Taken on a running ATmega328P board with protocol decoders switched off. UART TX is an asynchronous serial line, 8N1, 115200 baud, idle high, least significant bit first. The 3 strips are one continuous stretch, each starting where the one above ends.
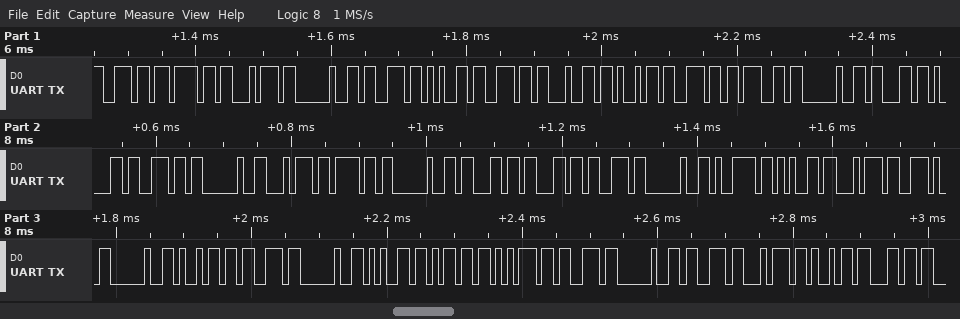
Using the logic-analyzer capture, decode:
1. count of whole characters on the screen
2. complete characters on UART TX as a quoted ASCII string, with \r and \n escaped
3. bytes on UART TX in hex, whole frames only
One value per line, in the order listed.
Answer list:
40
"not sending can to ccs yet. is emus stil"
6E 6F 74 20 73 65 6E 64 69 6E 67 20 63 61 6E 20 74 6F 20 63 63 73 20 79 65 74 2E 20 69 73 20 65 6D 75 73 20 73 74 69 6C
